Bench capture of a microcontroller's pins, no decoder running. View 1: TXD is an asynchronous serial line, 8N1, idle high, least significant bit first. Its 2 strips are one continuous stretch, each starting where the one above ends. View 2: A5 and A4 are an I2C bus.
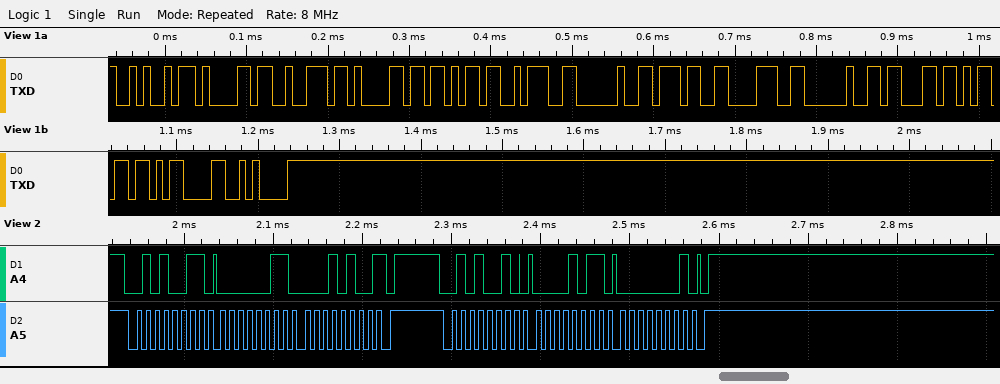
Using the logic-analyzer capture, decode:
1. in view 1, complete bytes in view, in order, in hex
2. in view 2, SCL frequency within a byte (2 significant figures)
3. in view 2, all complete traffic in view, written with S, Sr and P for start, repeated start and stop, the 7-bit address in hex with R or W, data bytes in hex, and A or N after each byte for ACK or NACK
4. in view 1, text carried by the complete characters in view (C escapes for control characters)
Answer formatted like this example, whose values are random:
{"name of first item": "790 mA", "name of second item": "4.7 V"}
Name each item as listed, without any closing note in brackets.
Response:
{"in view 1, complete bytes in view, in order, in hex": "0x4A 0x61 0x72 0x61 0x6B 0x3A 0x20 0x37 0x38 0x20 0x63 0x6D 0x0D 0x0A", "in view 2, SCL frequency within a byte": "100 kHz", "in view 2, all complete traffic in view, written with S, Sr and P for start, repeated start and stop, the 7-bit address in hex with R or W, data bytes in hex, and A or N after each byte for ACK or NACK": "S 29R A 03 A 14 N P S 29W A 0B A 01 A P", "in view 1, text carried by the complete characters in view": "\"Jarak: 78 cm\\r\\n\""}
